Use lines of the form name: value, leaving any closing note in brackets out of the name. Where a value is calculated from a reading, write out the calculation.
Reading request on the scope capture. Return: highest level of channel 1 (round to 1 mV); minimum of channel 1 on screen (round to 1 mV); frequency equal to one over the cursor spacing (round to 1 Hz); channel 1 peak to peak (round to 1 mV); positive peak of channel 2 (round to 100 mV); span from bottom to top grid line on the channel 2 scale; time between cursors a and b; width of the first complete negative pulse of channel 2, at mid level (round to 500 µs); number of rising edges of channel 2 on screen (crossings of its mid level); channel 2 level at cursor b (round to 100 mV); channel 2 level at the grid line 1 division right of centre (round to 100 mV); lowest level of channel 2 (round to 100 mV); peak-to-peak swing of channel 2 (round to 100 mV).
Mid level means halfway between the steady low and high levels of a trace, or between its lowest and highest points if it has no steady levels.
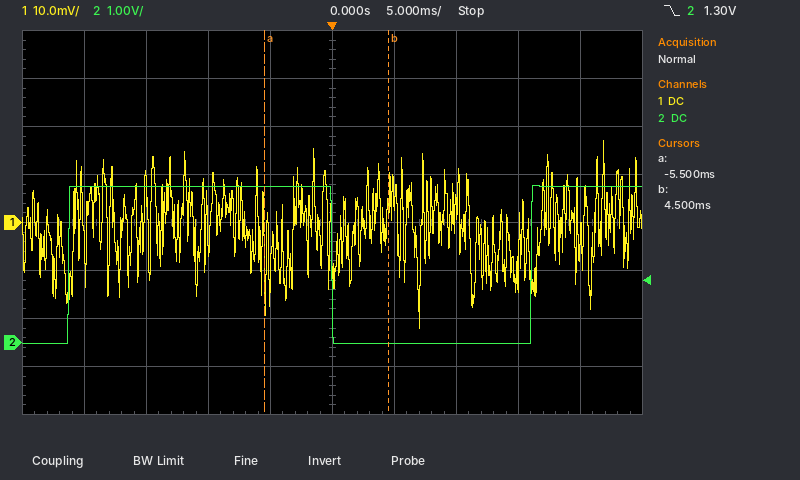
highest level of channel 1: 17 mV
minimum of channel 1 on screen: -22 mV
frequency equal to one over the cursor spacing: 1 / 10.0 ms ≈ 100 Hz
channel 1 peak to peak: 17 mV − (-22 mV) = 39 mV
positive peak of channel 2: 3.3 V
span from bottom to top grid line on the channel 2 scale: 8 V
time between cursors a and b: 4.5 ms − (-5.5 ms) = 10.0 ms
width of the first complete negative pulse of channel 2, at mid level: 16.0 ms
number of rising edges of channel 2 on screen: 2
channel 2 level at cursor b: 0.0 V
channel 2 level at the grid line 1 division right of centre: 0.0 V
lowest level of channel 2: 0.0 V
peak-to-peak swing of channel 2: 3.3 V − (0.0 V) = 3.3 V
